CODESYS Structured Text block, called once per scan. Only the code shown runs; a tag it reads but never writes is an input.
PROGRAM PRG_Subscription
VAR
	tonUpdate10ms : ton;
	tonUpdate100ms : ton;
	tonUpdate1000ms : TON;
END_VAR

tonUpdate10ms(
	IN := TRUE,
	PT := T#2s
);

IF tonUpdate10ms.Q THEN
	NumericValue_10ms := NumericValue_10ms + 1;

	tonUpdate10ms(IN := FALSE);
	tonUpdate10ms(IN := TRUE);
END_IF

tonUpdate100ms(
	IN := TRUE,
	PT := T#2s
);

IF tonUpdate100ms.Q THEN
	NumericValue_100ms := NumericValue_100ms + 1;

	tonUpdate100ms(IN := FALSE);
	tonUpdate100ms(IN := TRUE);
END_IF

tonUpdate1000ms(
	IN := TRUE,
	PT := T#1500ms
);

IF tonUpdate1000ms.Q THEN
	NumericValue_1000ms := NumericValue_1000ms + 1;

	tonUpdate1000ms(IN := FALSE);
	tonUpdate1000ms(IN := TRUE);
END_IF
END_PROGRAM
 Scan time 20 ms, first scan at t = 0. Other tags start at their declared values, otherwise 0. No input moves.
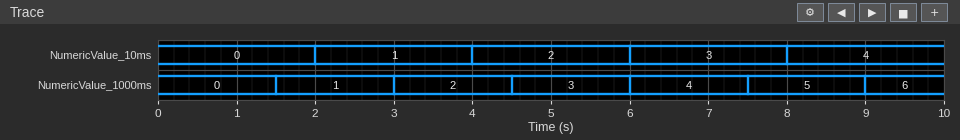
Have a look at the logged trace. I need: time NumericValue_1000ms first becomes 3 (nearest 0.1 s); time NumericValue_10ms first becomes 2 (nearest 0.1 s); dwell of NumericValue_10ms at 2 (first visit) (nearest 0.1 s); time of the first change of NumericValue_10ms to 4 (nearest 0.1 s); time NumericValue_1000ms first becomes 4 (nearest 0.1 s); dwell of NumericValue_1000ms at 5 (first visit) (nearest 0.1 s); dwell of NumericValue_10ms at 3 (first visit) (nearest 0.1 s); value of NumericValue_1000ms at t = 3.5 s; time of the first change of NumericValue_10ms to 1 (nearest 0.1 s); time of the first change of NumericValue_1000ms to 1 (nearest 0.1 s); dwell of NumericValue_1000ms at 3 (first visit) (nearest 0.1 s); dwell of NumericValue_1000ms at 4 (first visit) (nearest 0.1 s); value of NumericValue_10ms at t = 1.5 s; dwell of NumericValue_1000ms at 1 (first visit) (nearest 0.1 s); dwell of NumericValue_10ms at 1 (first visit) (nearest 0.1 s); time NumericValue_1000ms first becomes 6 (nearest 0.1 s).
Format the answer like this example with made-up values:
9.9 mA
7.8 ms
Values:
4.5 s
4.0 s
2.0 s
8.0 s
6.0 s
1.5 s
2.0 s
2
2.0 s
1.5 s
1.5 s
1.5 s
0
1.5 s
2.0 s
9.0 s
